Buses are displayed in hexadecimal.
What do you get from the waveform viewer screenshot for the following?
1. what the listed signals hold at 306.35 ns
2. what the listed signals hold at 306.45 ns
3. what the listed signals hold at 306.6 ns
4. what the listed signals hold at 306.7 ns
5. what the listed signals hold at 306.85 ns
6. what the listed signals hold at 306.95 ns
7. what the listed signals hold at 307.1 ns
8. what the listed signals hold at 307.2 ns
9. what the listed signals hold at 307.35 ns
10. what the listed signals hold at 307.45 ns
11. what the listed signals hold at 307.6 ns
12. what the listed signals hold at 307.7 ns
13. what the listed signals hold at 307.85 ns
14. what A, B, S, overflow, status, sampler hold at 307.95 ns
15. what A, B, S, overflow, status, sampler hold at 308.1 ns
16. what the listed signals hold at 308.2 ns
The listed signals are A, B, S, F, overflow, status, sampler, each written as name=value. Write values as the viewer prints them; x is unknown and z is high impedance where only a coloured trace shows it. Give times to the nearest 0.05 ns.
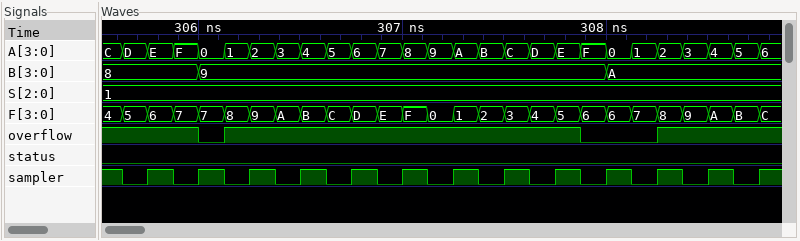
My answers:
A=2, B=9, S=1, F=9, overflow=1, status=0, sampler=1
A=3, B=9, S=1, F=A, overflow=1, status=0, sampler=0
A=4, B=9, S=1, F=B, overflow=1, status=0, sampler=1
A=5, B=9, S=1, F=C, overflow=1, status=0, sampler=0
A=6, B=9, S=1, F=D, overflow=1, status=0, sampler=1
A=7, B=9, S=1, F=E, overflow=1, status=0, sampler=0
A=8, B=9, S=1, F=F, overflow=1, status=0, sampler=1
A=9, B=9, S=1, F=0, overflow=1, status=0, sampler=0
A=A, B=9, S=1, F=1, overflow=1, status=0, sampler=1
A=B, B=9, S=1, F=2, overflow=1, status=0, sampler=0
A=C, B=9, S=1, F=3, overflow=1, status=0, sampler=1
A=D, B=9, S=1, F=4, overflow=1, status=0, sampler=0
A=E, B=9, S=1, F=5, overflow=1, status=0, sampler=1
A=F, B=9, S=1, overflow=0, status=0, sampler=0
A=0, B=A, S=1, overflow=0, status=0, sampler=1
A=1, B=A, S=1, F=7, overflow=0, status=0, sampler=0
